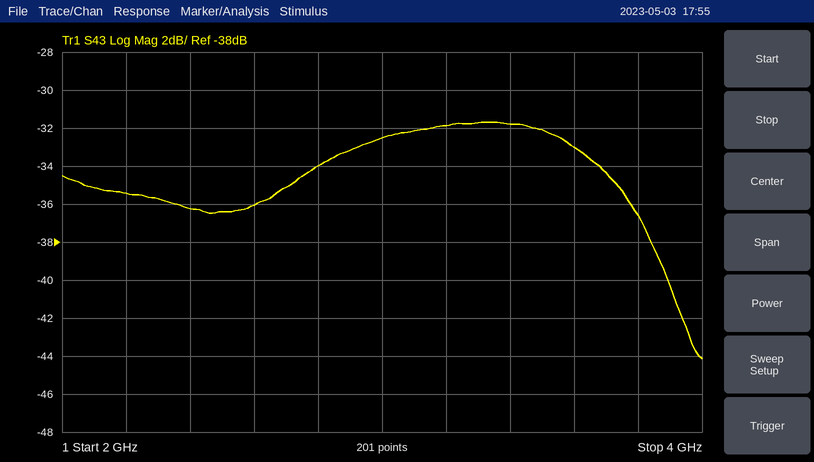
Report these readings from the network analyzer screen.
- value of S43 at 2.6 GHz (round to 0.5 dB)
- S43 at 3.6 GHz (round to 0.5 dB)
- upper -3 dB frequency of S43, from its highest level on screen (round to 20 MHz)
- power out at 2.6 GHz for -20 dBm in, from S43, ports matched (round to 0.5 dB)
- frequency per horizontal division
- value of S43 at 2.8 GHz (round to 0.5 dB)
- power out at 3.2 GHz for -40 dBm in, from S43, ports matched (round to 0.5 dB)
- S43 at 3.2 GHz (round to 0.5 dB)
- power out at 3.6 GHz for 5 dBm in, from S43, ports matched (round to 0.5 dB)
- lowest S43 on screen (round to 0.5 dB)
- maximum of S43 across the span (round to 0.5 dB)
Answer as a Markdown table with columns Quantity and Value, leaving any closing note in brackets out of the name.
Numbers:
| Quantity | Value |
|---|---|
| value of S43 at 2.6 GHz | -36.0 dB |
| S43 at 3.6 GHz | -33.0 dB |
| upper -3 dB frequency of S43, from its highest level on screen | 3.72 GHz |
| power out at 2.6 GHz for -20 dBm in, from S43, ports matched | -56.0 dBm |
| frequency per horizontal division | 200 MHz |
| value of S43 at 2.8 GHz | -34.0 dB |
| power out at 3.2 GHz for -40 dBm in, from S43, ports matched | -72.0 dBm |
| S43 at 3.2 GHz | -32.0 dB |
| power out at 3.6 GHz for 5 dBm in, from S43, ports matched | -28.0 dBm |
| lowest S43 on screen | -44.0 dB |
| maximum of S43 across the span | -31.5 dB |
